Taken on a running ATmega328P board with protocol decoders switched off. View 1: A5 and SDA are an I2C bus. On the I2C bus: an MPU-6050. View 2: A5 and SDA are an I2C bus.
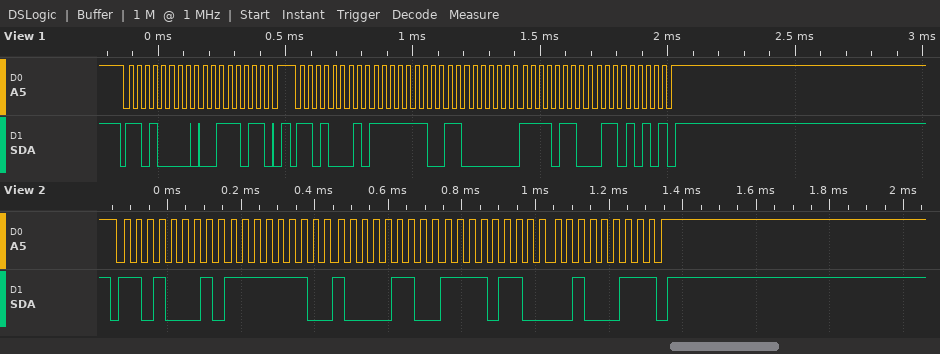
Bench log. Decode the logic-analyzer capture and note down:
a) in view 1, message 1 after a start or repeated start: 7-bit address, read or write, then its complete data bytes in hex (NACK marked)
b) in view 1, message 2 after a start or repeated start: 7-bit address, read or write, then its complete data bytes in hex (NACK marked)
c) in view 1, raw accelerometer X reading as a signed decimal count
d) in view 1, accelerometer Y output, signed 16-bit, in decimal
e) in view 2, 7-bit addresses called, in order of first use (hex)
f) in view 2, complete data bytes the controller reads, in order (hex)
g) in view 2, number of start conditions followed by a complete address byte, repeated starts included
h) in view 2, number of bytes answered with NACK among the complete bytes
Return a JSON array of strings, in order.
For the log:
["0x68 write: 3B", "0x68 read: FE C0 F6 6A NACK", "-320", "-2454", "0x68", "FE 86 F6 23", "1", "1"]
